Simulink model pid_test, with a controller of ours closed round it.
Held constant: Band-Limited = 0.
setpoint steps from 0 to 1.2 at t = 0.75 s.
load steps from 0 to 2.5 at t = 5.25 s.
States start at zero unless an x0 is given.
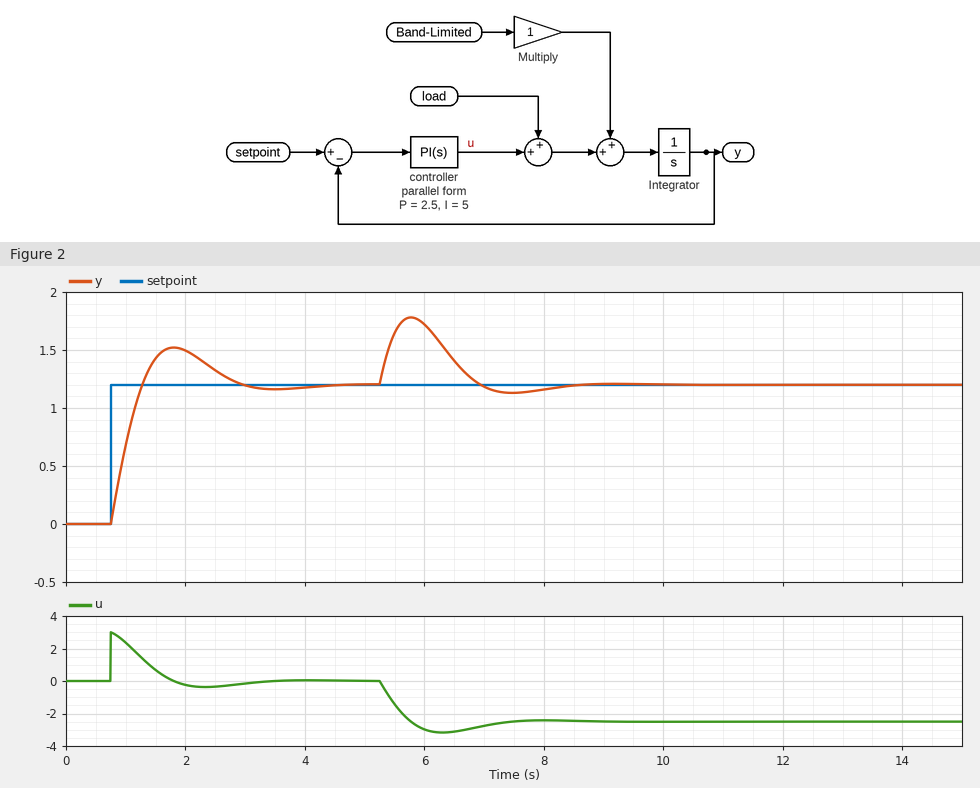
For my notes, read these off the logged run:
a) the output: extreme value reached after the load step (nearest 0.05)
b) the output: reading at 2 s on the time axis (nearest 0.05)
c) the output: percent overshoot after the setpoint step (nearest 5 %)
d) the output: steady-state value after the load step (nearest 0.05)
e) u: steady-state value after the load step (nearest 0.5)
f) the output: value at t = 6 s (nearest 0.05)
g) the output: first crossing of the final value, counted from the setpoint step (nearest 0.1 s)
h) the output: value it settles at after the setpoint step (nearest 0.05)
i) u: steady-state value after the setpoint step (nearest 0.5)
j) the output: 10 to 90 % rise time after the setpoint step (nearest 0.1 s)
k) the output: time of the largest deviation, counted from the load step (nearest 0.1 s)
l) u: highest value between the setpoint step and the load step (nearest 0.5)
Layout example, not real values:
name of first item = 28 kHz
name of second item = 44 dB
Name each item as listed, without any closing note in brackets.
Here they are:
the output: extreme value reached after the load step = 1.80
the output: reading at 2 s on the time axis = 1.50
the output: percent overshoot after the setpoint step = 25 %
the output: steady-state value after the load step = 1.20
u: steady-state value after the load step = -2.5
the output: value at t = 6 s = 1.70
the output: first crossing of the final value, counted from the setpoint step = 0.5 s
the output: value it settles at after the setpoint step = 1.20
u: steady-state value after the setpoint step = 0.0
the output: 10 to 90 % rise time after the setpoint step = 0.4 s
the output: time of the largest deviation, counted from the load step = 0.5 s
u: highest value between the setpoint step and the load step = 3.0
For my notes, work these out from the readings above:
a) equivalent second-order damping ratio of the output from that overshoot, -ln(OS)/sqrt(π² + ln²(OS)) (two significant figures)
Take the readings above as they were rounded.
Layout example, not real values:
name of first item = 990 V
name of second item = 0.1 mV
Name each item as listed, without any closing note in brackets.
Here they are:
equivalent second-order damping ratio of the output from that overshoot, -ln(OS)/sqrt(π² + ln²(OS)) = 0.40
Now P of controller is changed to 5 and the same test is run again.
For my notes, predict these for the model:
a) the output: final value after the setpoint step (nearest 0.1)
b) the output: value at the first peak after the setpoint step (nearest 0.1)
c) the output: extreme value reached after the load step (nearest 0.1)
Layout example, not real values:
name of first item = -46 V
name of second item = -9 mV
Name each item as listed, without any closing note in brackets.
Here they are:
the output: final value after the setpoint step = 1.2
the output: value at the first peak after the setpoint step = 1.3
the output: extreme value reached after the load step = 1.6
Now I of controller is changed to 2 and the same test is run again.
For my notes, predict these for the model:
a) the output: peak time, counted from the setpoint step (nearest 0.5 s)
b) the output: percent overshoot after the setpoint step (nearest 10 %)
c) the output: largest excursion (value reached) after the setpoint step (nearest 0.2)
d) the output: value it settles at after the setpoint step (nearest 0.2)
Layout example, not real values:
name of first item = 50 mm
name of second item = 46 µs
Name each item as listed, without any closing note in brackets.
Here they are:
the output: peak time, counted from the setpoint step = 1.5 s
the output: percent overshoot after the setpoint step = 20 %
the output: largest excursion (value reached) after the setpoint step = 1.4
the output: value it settles at after the setpoint step = 1.2
